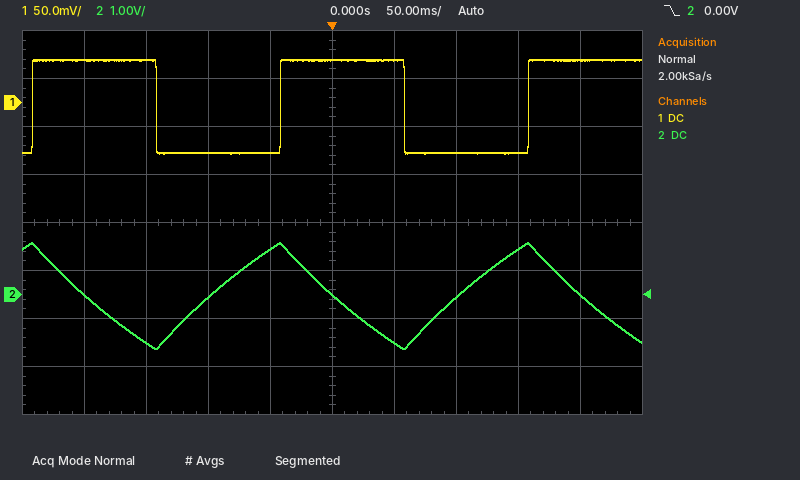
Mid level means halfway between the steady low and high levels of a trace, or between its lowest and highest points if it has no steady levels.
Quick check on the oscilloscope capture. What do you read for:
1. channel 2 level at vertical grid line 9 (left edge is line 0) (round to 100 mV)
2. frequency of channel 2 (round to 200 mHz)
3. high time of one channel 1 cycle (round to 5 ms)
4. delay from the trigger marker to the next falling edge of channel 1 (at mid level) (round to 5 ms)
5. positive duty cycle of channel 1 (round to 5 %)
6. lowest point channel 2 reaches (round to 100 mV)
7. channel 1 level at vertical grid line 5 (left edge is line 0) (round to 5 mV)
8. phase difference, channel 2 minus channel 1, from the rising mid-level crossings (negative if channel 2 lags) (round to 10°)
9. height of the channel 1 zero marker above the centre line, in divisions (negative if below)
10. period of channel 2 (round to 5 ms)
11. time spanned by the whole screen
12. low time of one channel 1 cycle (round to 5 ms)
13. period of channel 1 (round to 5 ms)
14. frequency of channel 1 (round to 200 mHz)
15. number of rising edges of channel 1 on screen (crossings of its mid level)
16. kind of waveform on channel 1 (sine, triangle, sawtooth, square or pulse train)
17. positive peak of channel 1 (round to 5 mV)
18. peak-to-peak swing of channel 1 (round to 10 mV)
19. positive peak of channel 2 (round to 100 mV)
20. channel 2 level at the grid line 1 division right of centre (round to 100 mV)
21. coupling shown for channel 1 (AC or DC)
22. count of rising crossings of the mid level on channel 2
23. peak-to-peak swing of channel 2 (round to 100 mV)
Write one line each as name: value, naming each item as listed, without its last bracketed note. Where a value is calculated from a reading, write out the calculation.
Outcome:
channel 2 level at vertical grid line 9 (left edge is line 0): 0.0 V
frequency of channel 2: 1 / 200 ms ≈ 5.0 Hz
high time of one channel 1 cycle: 100 ms
delay from the trigger marker to the next falling edge of channel 1 (at mid level): 60 ms
positive duty cycle of channel 1: 100 ms / 200 ms ≈ 50 %
lowest point channel 2 reaches: -1.1 V
channel 1 level at vertical grid line 5 (left edge is line 0): 45 mV
phase difference, channel 2 minus channel 1, from the rising mid-level crossings (negative if channel 2 lags): +100°
height of the channel 1 zero marker above the centre line, in divisions: +2.5 div
period of channel 2: 200 ms
time spanned by the whole screen: 500 ms
low time of one channel 1 cycle: 100 ms
period of channel 1: 200 ms
frequency of channel 1: 1 / 200 ms ≈ 5.0 Hz
number of rising edges of channel 1 on screen: 3
kind of waveform on channel 1: square
positive peak of channel 1: 45 mV
peak-to-peak swing of channel 1: 100 mV
positive peak of channel 2: 1.1 V
channel 2 level at the grid line 1 division right of centre: -1.0 V
coupling shown for channel 1: DC
count of rising crossings of the mid level on channel 2: 2
peak-to-peak swing of channel 2: 1.1 V − (-1.1 V) = 2.2 V
